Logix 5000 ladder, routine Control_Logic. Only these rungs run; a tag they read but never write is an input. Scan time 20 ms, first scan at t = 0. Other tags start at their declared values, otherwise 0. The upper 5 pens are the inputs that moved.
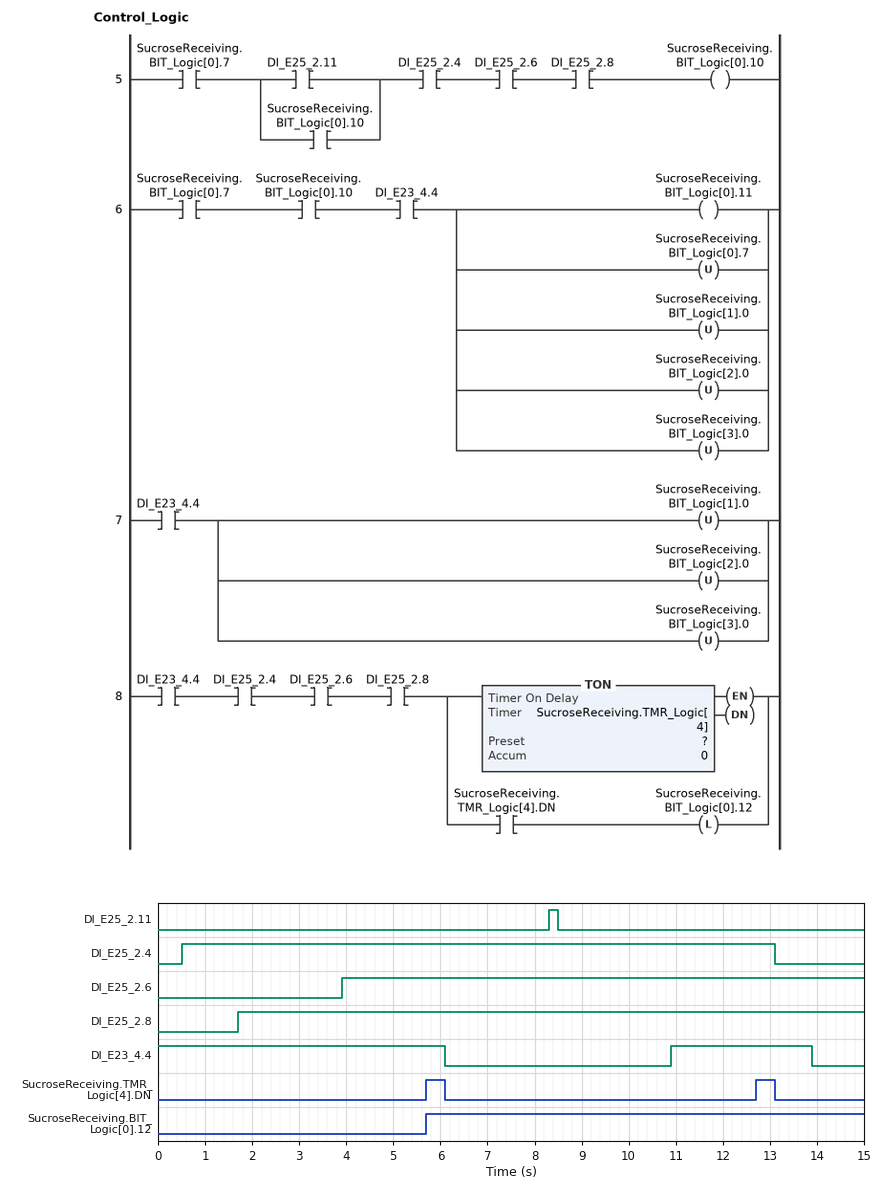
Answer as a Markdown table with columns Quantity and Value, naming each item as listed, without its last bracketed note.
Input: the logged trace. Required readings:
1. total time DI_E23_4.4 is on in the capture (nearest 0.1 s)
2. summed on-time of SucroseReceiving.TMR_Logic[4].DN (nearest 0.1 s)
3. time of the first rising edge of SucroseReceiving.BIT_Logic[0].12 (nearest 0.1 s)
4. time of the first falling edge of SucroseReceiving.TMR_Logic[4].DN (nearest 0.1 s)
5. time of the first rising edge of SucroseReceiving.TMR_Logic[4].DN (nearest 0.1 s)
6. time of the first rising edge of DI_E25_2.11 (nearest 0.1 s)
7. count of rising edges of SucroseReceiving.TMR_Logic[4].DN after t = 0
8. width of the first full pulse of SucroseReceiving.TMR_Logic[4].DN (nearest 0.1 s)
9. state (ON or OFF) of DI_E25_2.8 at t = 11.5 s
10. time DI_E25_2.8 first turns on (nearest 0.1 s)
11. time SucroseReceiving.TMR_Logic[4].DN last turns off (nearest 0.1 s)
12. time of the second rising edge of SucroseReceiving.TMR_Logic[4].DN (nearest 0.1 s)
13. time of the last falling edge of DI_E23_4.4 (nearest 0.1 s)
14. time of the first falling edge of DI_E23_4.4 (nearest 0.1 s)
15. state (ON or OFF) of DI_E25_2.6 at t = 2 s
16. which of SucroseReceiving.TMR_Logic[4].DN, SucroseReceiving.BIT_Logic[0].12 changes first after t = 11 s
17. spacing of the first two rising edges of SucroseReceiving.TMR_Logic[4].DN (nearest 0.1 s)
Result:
| Quantity | Value |
|---|---|
| total time DI_E23_4.4 is on in the capture | 9.1 s |
| summed on-time of SucroseReceiving.TMR_Logic[4].DN | 0.8 s |
| time of the first rising edge of SucroseReceiving.BIT_Logic[0].12 | 5.7 s |
| time of the first falling edge of SucroseReceiving.TMR_Logic[4].DN | 6.1 s |
| time of the first rising edge of SucroseReceiving.TMR_Logic[4].DN | 5.7 s |
| time of the first rising edge of DI_E25_2.11 | 8.3 s |
| count of rising edges of SucroseReceiving.TMR_Logic[4].DN after t = 0 | 2 |
| width of the first full pulse of SucroseReceiving.TMR_Logic[4].DN | 0.4 s |
| state (ON or OFF) of DI_E25_2.8 at t = 11.5 s | ON |
| time DI_E25_2.8 first turns on | 1.7 s |
| time SucroseReceiving.TMR_Logic[4].DN last turns off | 13.1 s |
| time of the second rising edge of SucroseReceiving.TMR_Logic[4].DN | 12.7 s |
| time of the last falling edge of DI_E23_4.4 | 13.9 s |
| time of the first falling edge of DI_E23_4.4 | 6.1 s |
| state (ON or OFF) of DI_E25_2.6 at t = 2 s | OFF |
| which of SucroseReceiving.TMR_Logic[4].DN, SucroseReceiving.BIT_Logic[0].12 changes first after t = 11 s | SucroseReceiving.TMR_Logic[4].DN |
| spacing of the first two rising edges of SucroseReceiving.TMR_Logic[4].DN | 7.0 s |
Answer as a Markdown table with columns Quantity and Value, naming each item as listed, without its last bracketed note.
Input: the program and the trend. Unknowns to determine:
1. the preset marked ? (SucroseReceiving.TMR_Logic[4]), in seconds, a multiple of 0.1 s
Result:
| Quantity | Value |
|---|---|
| the preset marked ? (SucroseReceiving.TMR_Logic[4]), in seconds, a multiple of 0.1 s | 1.8 s |
